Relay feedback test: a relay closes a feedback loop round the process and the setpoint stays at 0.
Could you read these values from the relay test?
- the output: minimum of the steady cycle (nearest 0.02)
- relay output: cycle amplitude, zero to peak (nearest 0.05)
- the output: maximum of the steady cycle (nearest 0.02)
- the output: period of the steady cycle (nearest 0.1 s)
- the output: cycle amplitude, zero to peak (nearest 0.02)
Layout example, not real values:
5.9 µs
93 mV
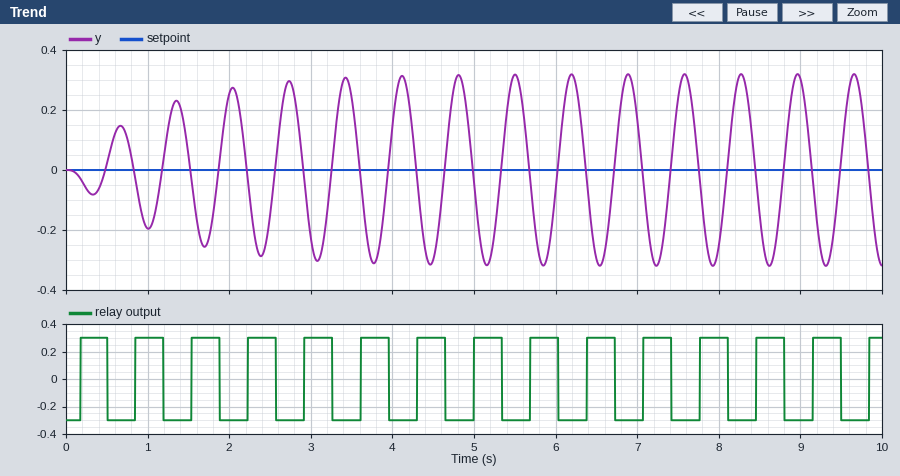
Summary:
-0.32
0.30
0.32
0.7 s
0.32
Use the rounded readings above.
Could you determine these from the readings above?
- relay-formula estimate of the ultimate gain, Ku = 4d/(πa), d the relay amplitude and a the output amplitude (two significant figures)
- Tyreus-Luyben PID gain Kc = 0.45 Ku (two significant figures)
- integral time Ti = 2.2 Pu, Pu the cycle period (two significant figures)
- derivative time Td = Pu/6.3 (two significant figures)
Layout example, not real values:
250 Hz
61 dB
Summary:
1.2
0.54
1.5 s
0.11 s
